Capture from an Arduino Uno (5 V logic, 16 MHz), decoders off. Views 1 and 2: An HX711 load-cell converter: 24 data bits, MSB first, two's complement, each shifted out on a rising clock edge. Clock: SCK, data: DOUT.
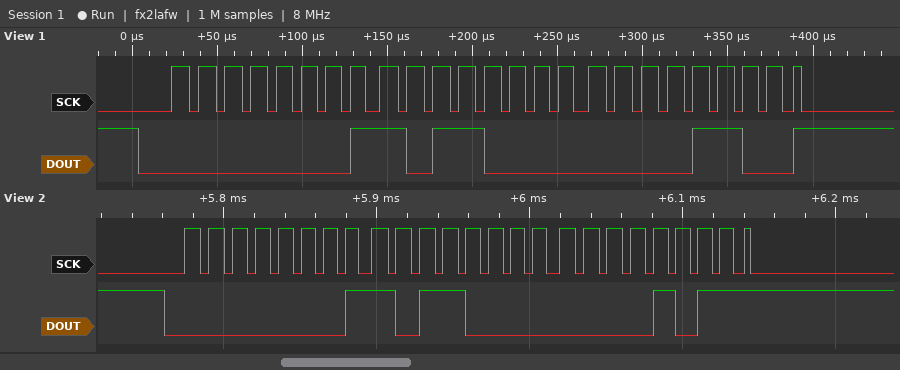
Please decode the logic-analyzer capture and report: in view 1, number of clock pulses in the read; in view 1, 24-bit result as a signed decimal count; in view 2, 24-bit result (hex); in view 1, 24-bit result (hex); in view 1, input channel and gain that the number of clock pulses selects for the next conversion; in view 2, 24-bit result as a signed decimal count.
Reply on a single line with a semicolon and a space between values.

25; 110604; 0x01B00B; 0x01B00C; channel A, gain 128; 110603
